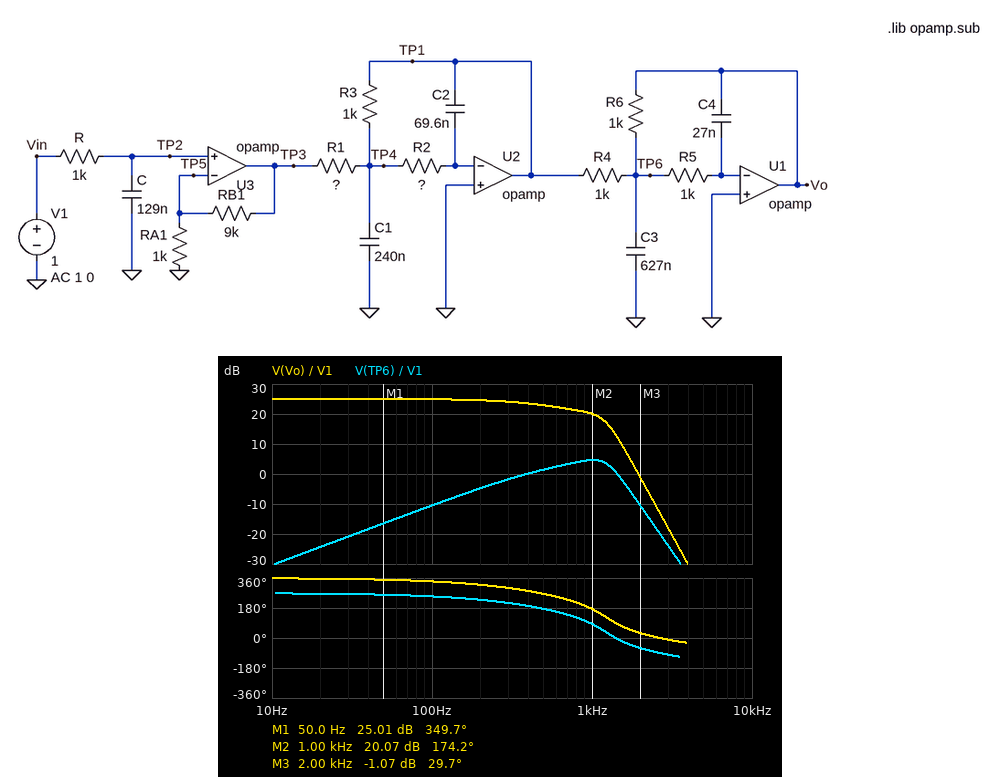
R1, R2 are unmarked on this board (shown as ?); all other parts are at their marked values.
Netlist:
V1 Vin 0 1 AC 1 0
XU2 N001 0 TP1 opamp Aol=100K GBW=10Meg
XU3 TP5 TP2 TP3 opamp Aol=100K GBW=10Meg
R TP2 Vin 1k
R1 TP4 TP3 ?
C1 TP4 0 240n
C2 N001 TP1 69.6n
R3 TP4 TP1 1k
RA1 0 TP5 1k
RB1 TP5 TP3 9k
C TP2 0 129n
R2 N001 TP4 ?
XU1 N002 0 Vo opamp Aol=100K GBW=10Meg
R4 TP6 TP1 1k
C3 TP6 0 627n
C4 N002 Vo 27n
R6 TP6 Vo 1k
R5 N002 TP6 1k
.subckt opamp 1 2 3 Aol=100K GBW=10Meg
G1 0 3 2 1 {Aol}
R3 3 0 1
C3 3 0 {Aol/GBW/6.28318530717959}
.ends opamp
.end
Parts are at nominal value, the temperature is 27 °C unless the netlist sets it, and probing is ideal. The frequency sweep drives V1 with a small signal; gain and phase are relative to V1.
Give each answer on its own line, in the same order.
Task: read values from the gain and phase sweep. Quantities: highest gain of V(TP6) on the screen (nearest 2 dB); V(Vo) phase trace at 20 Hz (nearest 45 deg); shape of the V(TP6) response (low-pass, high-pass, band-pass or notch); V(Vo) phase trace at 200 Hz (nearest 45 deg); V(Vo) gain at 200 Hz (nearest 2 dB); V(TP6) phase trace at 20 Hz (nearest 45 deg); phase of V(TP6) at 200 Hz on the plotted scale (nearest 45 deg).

4 dB
360 deg
band-pass
315 deg
24 dB
270 deg
225 deg
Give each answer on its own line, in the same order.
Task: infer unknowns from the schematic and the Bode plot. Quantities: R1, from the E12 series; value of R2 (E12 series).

560 Ω
1.5 kΩ
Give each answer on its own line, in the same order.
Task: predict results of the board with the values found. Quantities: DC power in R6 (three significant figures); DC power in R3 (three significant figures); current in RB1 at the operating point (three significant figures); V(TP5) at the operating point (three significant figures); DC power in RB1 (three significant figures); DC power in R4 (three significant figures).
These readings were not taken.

319 mW
319 mW
1.00 mA
1.00 V
9.00 mW
319 mW
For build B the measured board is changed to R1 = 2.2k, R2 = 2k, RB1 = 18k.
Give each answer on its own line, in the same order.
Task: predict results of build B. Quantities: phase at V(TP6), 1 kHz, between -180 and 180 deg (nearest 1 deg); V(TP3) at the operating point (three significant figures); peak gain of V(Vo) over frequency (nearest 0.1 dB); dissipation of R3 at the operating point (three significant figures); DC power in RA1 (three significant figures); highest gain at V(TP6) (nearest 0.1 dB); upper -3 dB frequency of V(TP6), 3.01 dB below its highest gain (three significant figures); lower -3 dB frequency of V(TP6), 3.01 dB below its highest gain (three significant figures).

73 deg
19.0 V
18.7 dB
74.6 mW
1.00 mW
0.7 dB
1.30 kHz
536 Hz
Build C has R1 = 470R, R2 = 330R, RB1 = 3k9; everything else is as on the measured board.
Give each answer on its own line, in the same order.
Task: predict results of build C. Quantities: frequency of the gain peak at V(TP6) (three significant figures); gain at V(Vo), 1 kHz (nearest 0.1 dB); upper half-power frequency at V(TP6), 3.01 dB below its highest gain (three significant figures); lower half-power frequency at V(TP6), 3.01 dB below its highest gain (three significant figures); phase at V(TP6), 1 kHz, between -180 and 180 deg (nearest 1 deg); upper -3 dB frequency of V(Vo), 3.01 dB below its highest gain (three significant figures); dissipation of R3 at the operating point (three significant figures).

1.12 kHz
21.0 dB
1.45 kHz
756 Hz
125 deg
1.30 kHz
109 mW
